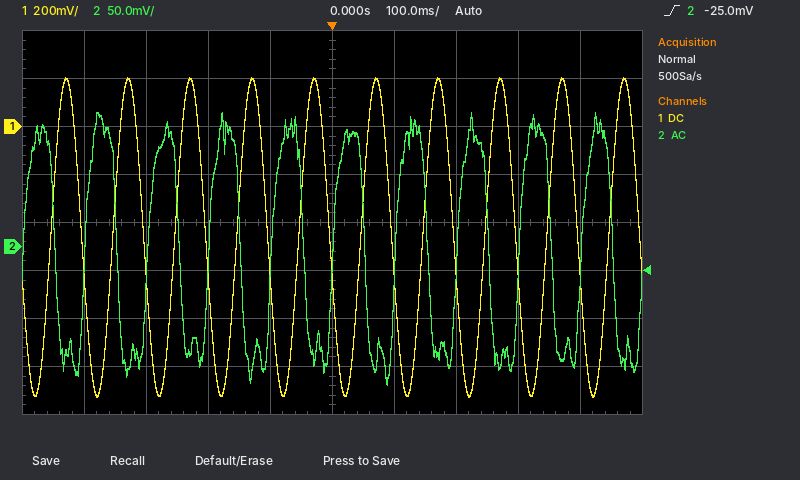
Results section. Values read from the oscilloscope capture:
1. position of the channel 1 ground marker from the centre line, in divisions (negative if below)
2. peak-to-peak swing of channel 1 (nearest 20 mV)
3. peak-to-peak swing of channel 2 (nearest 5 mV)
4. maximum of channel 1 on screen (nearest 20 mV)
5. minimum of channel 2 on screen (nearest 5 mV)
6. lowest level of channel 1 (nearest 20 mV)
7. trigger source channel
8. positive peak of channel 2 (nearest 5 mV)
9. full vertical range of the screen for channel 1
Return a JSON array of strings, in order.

["+2.0 div", "1.32 V", "285 mV", "200 mV", "-145 mV", "-1.12 V", "channel 2", "140 mV", "1.6 V"]
